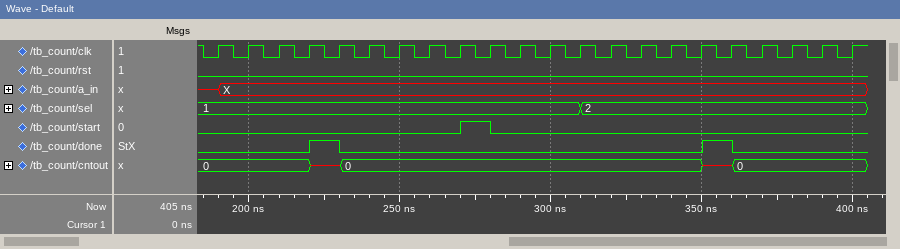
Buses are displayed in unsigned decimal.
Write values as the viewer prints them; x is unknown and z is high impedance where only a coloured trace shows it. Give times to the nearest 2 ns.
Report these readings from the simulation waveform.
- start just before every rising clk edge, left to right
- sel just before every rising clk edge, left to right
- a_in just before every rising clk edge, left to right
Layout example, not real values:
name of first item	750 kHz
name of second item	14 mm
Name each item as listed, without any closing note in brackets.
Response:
start just before every rising clk edge, left to right	0 0 0 0 0 0 0 0 0 1 0 0 0 0 0 0 0 0 0 0 0 0
sel just before every rising clk edge, left to right	1, 1, 1, 1, 1, 1, 1, 1, 1, 1, 1, 1, 1, 2, 2, 2, 2, 2, 2, 2, 2, 2
a_in just before every rising clk edge, left to right	x, X, X, X, X, X, X, X, X, X, X, X, X, X, X, X, X, X, X, X, X, X
